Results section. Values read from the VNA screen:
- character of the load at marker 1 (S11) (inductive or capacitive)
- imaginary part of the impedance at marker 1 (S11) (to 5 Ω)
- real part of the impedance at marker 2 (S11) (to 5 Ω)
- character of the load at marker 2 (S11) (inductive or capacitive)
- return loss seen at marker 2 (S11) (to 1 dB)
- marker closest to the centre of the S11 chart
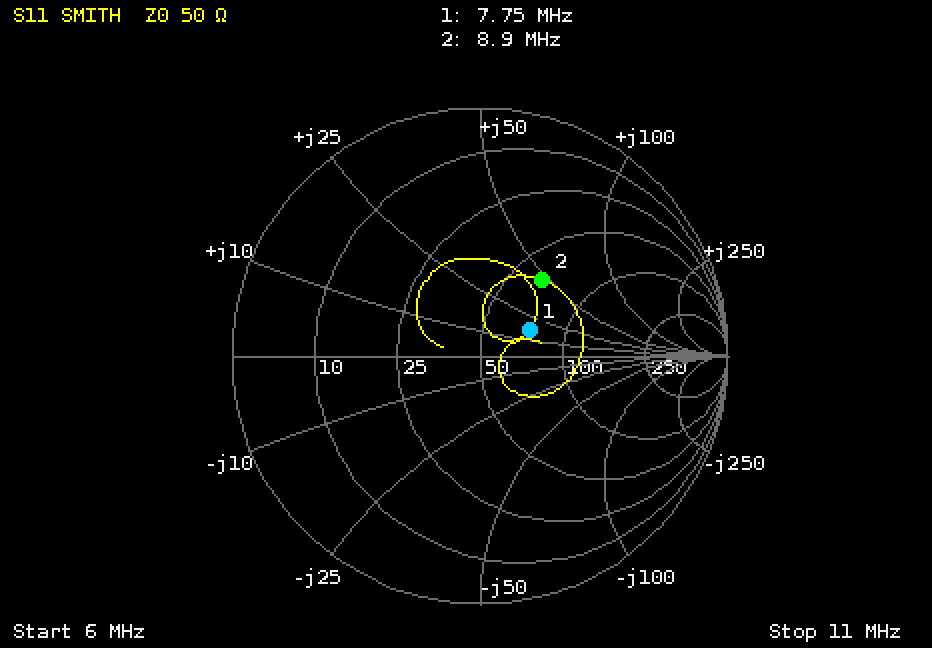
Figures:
inductive
+15 Ω
65 Ω
inductive
8 dB
marker 1
